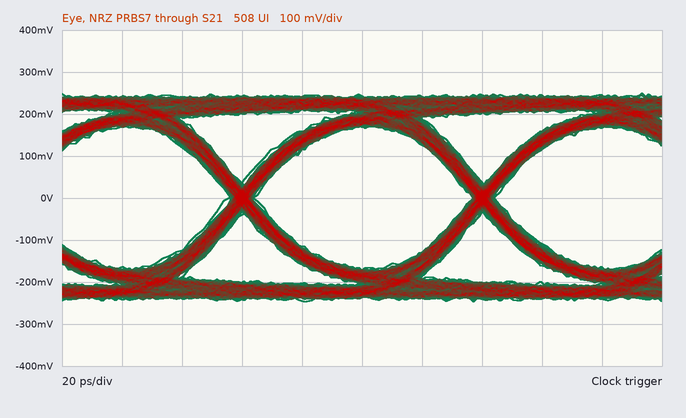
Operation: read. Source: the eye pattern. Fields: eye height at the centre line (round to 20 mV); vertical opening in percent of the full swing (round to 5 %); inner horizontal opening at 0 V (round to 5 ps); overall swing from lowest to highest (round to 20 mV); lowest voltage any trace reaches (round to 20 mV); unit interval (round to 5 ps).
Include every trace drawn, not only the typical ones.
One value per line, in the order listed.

340 mV
70 %
75 ps
500 mV
-240 mV
80 ps
